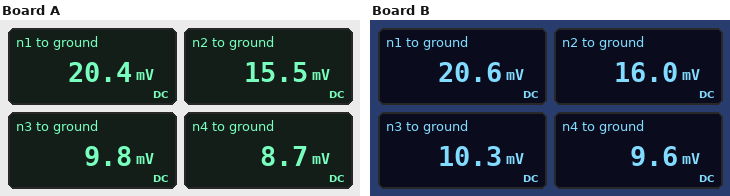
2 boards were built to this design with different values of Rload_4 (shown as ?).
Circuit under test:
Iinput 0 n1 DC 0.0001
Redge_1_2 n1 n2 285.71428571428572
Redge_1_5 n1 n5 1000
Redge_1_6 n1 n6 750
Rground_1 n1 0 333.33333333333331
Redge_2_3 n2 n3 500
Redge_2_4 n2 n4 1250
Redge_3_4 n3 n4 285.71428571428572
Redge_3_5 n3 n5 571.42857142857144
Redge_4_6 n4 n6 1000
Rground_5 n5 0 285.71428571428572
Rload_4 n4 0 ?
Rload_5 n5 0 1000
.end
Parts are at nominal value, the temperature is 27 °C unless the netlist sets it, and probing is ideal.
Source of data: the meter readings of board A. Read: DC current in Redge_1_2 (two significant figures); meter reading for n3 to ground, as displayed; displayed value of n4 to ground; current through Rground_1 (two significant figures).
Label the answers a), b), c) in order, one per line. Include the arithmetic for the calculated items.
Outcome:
a) (20.4 mV - 15.5 mV) / 285.7 Ω = 17 µA
b) 9.8 mV
c) 8.7 mV
d) (20.4 mV) / 333.3 Ω = 61 µA
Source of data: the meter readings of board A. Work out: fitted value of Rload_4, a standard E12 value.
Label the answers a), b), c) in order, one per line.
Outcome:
a) 560 Ω
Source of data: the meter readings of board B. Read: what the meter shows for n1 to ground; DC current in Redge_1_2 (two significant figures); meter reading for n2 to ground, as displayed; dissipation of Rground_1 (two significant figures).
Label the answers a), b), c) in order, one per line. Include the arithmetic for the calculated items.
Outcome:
a) 20.6 mV
b) (20.6 mV - 16 mV) / 285.7 Ω = 16 µA
c) 16.0 mV
d) (20.6 mV)^2 / 333.3 Ω = 1.3 µW
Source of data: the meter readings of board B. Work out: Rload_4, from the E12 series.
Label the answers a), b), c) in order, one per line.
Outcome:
a) 680 Ω
